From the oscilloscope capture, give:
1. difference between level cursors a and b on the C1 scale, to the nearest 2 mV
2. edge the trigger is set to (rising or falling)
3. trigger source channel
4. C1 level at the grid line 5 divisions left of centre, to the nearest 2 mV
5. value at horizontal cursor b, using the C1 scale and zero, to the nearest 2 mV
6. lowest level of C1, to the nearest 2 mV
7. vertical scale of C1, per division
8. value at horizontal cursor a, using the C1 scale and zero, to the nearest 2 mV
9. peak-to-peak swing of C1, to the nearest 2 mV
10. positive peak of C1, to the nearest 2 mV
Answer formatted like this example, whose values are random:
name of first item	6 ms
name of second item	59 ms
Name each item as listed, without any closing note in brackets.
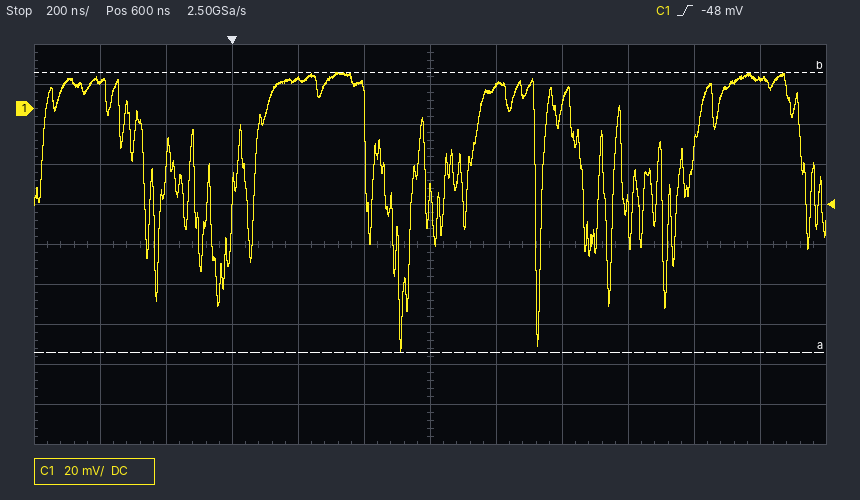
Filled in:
difference between level cursors a and b on the C1 scale, to the nearest 2 mV	140 mV
edge the trigger is set to	rising
trigger source channel	C1
C1 level at the grid line 5 divisions left of centre, to the nearest 2 mV	14 mV
value at horizontal cursor b, using the C1 scale and zero, to the nearest 2 mV	18 mV
lowest level of C1, to the nearest 2 mV	-122 mV
vertical scale of C1, per division	20 mV
value at horizontal cursor a, using the C1 scale and zero, to the nearest 2 mV	-122 mV
peak-to-peak swing of C1, to the nearest 2 mV	140 mV
positive peak of C1, to the nearest 2 mV	18 mV
